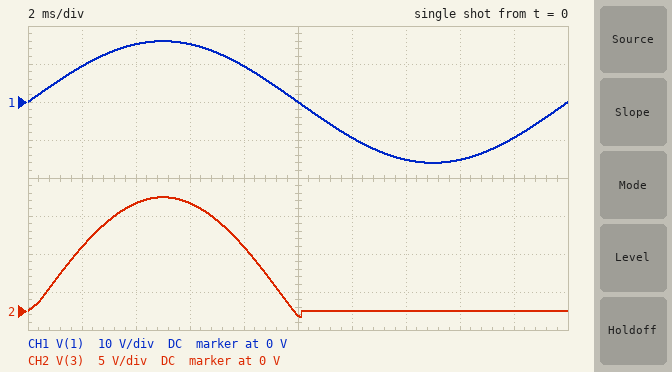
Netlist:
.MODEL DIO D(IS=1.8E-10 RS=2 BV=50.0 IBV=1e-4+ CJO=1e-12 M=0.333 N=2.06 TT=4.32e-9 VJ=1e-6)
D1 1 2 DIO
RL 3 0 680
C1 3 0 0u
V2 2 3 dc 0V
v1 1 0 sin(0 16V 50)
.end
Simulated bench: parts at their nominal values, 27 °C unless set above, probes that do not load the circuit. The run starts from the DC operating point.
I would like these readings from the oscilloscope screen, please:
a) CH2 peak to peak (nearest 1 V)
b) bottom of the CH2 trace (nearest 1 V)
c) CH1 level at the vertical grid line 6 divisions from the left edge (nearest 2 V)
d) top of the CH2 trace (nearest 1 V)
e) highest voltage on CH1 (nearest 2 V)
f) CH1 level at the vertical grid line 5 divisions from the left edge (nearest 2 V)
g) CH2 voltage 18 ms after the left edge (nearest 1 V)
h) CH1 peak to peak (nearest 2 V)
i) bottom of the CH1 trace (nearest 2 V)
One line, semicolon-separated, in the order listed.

16 V; -1 V; -10 V; 15 V; 16 V; 0 V; 0 V; 32 V; -16 V
